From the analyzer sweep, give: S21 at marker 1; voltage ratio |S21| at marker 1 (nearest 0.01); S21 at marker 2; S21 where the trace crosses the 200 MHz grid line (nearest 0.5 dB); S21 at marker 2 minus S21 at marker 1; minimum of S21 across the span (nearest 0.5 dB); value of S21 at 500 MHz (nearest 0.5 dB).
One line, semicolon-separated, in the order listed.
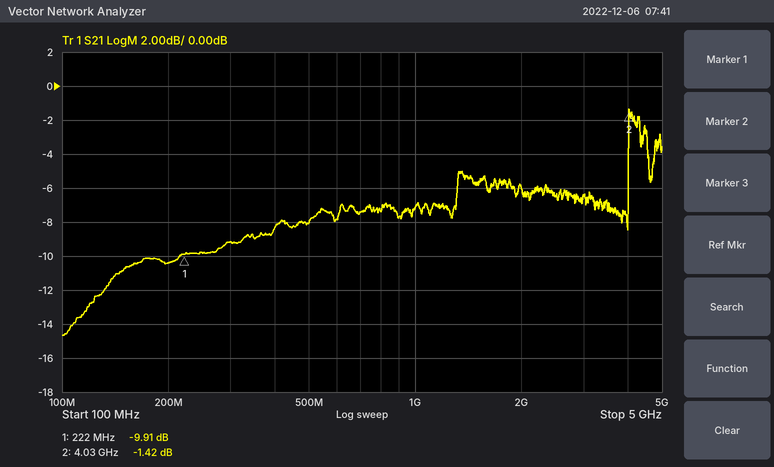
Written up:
-9.91 dB; 0.32; -1.42 dB; -10.5 dB; 8.49 dB; -14.5 dB; -8.0 dB
